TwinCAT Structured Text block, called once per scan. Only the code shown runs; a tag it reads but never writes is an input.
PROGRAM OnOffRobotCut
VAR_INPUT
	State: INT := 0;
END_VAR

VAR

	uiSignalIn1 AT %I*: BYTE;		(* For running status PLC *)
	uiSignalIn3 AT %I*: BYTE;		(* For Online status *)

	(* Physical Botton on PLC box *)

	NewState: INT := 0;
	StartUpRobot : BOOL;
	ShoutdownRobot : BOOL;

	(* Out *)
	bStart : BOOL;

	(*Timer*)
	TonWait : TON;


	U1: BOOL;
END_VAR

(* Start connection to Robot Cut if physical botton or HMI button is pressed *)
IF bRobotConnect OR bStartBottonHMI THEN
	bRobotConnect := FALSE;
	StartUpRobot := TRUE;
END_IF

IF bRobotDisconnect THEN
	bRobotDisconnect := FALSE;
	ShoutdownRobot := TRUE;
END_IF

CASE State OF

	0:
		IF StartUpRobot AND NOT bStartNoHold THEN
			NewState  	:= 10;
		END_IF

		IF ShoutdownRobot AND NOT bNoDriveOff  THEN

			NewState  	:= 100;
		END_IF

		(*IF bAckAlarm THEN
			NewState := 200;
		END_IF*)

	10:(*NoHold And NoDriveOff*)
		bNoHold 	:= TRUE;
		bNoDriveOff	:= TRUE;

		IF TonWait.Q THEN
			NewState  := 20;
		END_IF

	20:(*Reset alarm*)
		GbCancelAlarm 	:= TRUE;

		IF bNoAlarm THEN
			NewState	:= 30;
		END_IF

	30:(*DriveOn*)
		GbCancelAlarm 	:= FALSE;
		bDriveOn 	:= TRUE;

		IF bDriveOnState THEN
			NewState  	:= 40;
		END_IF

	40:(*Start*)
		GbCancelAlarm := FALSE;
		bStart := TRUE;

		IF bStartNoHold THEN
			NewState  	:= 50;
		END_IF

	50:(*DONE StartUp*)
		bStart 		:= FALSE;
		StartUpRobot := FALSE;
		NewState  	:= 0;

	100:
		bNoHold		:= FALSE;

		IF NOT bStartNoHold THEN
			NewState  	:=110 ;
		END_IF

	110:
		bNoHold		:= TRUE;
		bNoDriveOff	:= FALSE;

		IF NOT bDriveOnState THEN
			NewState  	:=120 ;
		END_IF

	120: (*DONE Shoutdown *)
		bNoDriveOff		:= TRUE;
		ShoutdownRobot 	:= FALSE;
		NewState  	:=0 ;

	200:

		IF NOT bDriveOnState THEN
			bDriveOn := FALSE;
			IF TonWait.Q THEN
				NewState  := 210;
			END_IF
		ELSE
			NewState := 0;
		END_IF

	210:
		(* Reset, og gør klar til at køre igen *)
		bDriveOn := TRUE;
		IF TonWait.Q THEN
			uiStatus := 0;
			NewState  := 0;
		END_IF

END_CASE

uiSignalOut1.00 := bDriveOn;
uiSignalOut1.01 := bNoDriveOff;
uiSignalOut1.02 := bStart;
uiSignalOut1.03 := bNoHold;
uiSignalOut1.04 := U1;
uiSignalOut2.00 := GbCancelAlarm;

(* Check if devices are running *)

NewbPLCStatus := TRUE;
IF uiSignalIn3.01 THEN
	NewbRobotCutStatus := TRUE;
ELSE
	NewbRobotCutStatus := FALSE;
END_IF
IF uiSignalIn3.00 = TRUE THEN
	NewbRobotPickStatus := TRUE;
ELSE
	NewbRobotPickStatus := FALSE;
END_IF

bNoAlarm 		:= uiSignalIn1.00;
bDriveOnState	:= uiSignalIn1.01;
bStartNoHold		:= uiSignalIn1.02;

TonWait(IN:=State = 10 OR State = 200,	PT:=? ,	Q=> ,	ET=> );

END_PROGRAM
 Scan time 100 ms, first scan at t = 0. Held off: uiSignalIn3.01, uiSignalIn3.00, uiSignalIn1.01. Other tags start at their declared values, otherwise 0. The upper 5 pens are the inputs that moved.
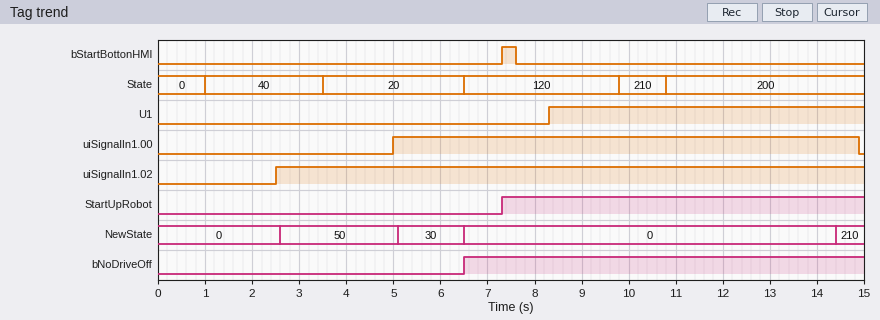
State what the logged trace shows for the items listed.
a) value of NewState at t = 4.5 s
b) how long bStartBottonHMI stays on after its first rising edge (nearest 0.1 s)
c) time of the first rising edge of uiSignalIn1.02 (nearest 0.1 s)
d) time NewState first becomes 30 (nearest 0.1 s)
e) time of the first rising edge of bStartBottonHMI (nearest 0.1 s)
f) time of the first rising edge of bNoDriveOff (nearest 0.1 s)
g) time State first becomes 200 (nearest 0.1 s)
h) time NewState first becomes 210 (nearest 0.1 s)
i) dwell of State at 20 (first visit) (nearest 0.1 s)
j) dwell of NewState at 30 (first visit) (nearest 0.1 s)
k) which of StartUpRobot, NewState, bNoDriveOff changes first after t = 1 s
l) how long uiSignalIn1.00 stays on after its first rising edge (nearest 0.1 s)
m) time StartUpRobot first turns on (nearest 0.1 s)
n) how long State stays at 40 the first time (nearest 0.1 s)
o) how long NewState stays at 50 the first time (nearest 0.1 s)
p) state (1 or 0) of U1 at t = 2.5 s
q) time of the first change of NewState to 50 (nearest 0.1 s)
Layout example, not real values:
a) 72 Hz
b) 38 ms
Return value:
a) 50
b) 0.3 s
c) 2.5 s
d) 5.1 s
e) 7.3 s
f) 6.5 s
g) 10.8 s
h) 14.4 s
i) 3.0 s
j) 1.4 s
k) NewState
l) 9.9 s
m) 7.3 s
n) 2.5 s
o) 2.5 s
p) 0
q) 2.6 s
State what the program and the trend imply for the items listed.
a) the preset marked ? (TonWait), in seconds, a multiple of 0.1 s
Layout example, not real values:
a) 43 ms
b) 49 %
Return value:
a) 3.5 s
